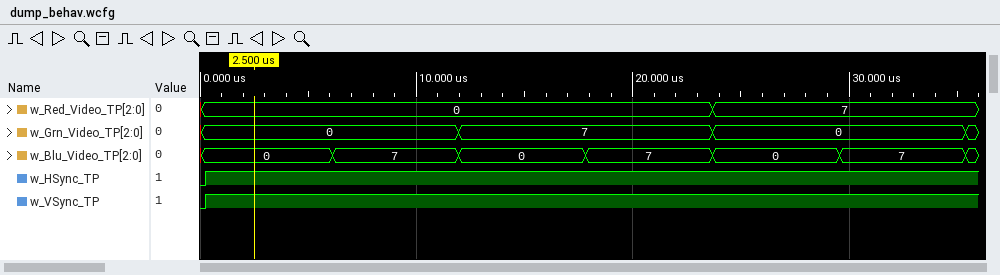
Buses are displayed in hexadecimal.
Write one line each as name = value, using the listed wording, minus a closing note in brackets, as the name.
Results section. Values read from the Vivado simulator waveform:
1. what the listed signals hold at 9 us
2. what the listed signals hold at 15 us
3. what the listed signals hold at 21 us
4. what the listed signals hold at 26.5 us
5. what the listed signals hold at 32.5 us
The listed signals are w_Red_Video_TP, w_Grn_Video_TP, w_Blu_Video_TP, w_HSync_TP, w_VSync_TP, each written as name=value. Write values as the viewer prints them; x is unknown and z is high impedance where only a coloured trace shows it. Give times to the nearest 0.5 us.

what the listed signals hold at 9 us = w_Red_Video_TP=0, w_Grn_Video_TP=0, w_Blu_Video_TP=7, w_HSync_TP=1, w_VSync_TP=1
what the listed signals hold at 15 us = w_Red_Video_TP=0, w_Grn_Video_TP=7, w_Blu_Video_TP=0, w_HSync_TP=1, w_VSync_TP=1
what the listed signals hold at 21 us = w_Red_Video_TP=0, w_Grn_Video_TP=7, w_Blu_Video_TP=7, w_HSync_TP=1, w_VSync_TP=1
what the listed signals hold at 26.5 us = w_Red_Video_TP=7, w_Grn_Video_TP=0, w_Blu_Video_TP=0, w_HSync_TP=1, w_VSync_TP=1
what the listed signals hold at 32.5 us = w_Red_Video_TP=7, w_Grn_Video_TP=0, w_Blu_Video_TP=7, w_HSync_TP=1, w_VSync_TP=1
